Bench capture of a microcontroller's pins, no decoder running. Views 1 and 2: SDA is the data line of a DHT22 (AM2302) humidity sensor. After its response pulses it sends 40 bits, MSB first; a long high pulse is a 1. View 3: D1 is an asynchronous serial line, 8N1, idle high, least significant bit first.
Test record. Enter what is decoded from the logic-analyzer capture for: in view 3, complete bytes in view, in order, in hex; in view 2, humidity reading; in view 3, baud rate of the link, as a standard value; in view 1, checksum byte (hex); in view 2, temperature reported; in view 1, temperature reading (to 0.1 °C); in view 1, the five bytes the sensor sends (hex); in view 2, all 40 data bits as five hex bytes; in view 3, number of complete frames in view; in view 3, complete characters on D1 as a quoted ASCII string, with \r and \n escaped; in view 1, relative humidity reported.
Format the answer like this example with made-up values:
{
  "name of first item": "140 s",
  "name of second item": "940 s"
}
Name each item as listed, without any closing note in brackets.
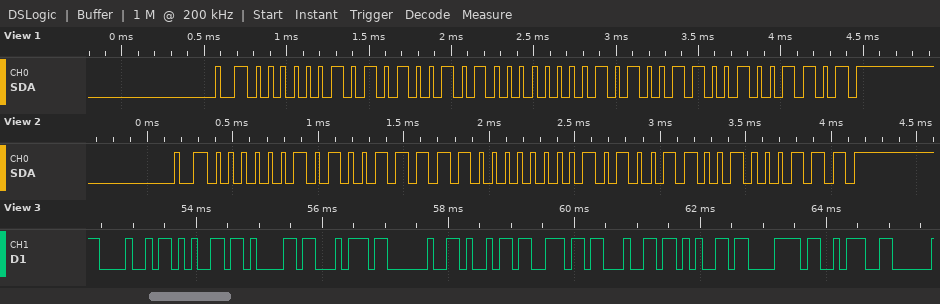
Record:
{
  "in view 3, complete bytes in view, in order, in hex": "48 65 61 74 20 69 6E 64 65 78 3A",
  "in view 2, humidity reading": "67.1 %",
  "in view 3, baud rate of the link, as a standard value": "9600 baud",
  "in view 1, checksum byte": "0x4D",
  "in view 2, temperature reported": "16.6 °C",
  "in view 1, temperature reading": "16.6 °C",
  "in view 1, the five bytes the sensor sends": "02 A5 00 A6 4D",
  "in view 2, all 40 data bits as five hex bytes": "02 9F 00 A6 47",
  "in view 3, number of complete frames in view": "11",
  "in view 3, complete characters on D1 as a quoted ASCII string, with \\r and \\n escaped": "\"Heat index:\"",
  "in view 1, relative humidity reported": "67.7 %"
}
